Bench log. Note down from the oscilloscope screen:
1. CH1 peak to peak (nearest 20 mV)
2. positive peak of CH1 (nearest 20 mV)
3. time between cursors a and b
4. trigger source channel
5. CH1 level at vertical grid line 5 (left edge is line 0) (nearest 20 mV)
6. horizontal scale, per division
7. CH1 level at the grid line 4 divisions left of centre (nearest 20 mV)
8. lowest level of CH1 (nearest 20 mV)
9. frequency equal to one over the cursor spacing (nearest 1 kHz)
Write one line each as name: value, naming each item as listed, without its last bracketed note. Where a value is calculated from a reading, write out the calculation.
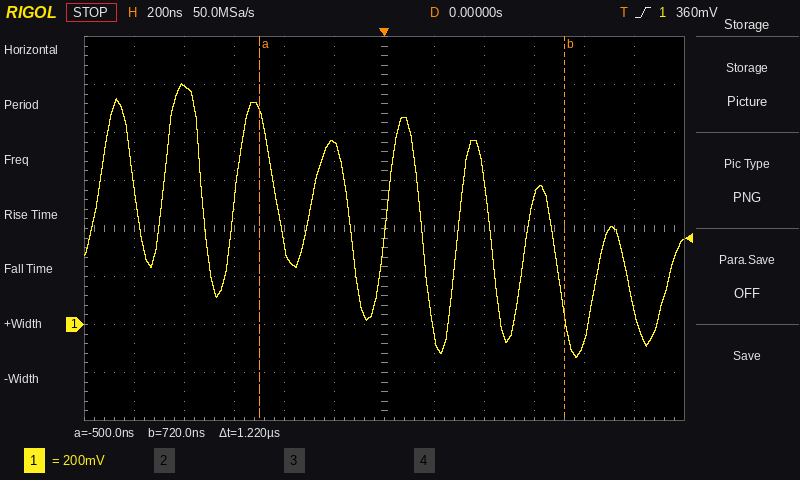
CH1 peak to peak: 1.00 V − (-140 mV) = 1.14 V
positive peak of CH1: 1.00 V
time between cursors a and b: 1.22 µs
trigger source channel: CH1
CH1 level at vertical grid line 5 (left edge is line 0): 760 mV
horizontal scale, per division: 200 ns
CH1 level at the grid line 4 divisions left of centre: 1.00 V
lowest level of CH1: -140 mV
frequency equal to one over the cursor spacing: 1 / 1.22 µs ≈ 820 kHz
